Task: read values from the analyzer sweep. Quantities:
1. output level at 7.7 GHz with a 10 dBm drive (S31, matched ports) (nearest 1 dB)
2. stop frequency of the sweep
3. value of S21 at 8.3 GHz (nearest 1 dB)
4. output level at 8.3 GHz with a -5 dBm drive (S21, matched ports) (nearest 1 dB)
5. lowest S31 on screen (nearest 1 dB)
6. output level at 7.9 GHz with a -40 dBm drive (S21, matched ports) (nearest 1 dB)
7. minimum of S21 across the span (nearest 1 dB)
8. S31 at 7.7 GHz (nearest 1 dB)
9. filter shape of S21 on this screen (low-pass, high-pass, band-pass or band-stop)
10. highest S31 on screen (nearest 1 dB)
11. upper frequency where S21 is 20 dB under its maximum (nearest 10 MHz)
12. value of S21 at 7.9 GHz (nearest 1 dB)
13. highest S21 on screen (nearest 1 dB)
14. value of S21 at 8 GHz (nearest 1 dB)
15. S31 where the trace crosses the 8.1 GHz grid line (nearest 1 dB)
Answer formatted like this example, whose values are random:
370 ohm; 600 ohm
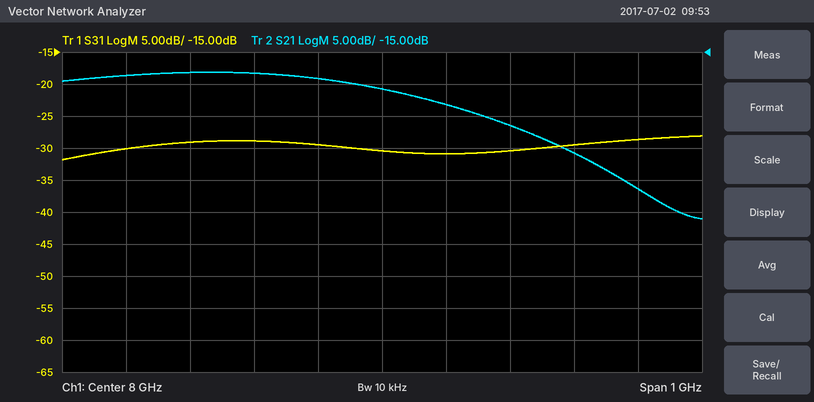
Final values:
-19 dBm; 8.5 GHz; -31 dB; -36 dBm; -32 dB; -59 dBm; -41 dB; -29 dB; low-pass; -28 dB; 8.43 GHz; -19 dB; -18 dB; -21 dB; -31 dB
